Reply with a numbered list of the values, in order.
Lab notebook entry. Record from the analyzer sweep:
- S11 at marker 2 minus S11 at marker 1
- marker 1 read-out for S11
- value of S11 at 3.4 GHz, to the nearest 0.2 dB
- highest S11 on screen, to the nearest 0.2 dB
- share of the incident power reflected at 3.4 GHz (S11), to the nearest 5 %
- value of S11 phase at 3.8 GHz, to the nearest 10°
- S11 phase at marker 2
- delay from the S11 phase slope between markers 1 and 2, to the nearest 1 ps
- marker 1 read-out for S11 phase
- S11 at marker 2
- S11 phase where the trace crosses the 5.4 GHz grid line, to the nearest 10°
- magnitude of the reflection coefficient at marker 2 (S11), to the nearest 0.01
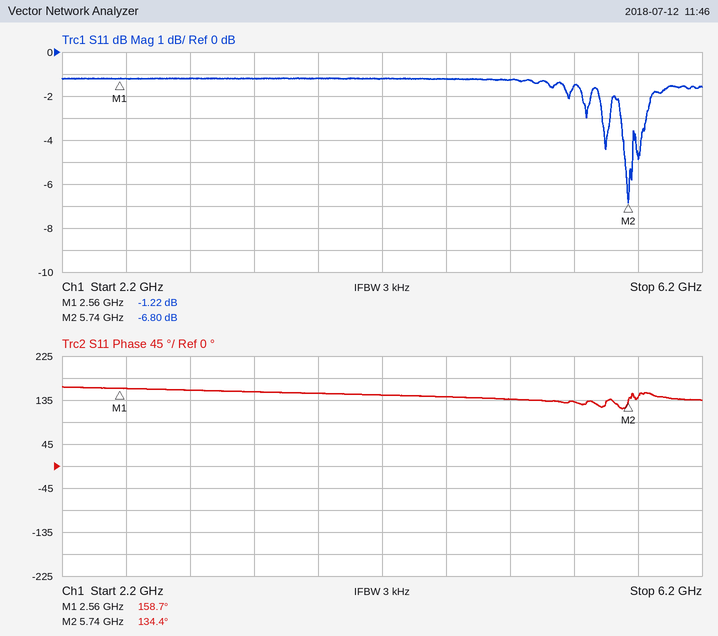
1. -5.58 dB
2. -1.22 dB
3. -1.2 dB
4. -1.2 dB
5. 75 %
6. 150°
7. 134.4°
8. 21 ps
9. 158.7°
10. -6.80 dB
11. 130°
12. 0.46
